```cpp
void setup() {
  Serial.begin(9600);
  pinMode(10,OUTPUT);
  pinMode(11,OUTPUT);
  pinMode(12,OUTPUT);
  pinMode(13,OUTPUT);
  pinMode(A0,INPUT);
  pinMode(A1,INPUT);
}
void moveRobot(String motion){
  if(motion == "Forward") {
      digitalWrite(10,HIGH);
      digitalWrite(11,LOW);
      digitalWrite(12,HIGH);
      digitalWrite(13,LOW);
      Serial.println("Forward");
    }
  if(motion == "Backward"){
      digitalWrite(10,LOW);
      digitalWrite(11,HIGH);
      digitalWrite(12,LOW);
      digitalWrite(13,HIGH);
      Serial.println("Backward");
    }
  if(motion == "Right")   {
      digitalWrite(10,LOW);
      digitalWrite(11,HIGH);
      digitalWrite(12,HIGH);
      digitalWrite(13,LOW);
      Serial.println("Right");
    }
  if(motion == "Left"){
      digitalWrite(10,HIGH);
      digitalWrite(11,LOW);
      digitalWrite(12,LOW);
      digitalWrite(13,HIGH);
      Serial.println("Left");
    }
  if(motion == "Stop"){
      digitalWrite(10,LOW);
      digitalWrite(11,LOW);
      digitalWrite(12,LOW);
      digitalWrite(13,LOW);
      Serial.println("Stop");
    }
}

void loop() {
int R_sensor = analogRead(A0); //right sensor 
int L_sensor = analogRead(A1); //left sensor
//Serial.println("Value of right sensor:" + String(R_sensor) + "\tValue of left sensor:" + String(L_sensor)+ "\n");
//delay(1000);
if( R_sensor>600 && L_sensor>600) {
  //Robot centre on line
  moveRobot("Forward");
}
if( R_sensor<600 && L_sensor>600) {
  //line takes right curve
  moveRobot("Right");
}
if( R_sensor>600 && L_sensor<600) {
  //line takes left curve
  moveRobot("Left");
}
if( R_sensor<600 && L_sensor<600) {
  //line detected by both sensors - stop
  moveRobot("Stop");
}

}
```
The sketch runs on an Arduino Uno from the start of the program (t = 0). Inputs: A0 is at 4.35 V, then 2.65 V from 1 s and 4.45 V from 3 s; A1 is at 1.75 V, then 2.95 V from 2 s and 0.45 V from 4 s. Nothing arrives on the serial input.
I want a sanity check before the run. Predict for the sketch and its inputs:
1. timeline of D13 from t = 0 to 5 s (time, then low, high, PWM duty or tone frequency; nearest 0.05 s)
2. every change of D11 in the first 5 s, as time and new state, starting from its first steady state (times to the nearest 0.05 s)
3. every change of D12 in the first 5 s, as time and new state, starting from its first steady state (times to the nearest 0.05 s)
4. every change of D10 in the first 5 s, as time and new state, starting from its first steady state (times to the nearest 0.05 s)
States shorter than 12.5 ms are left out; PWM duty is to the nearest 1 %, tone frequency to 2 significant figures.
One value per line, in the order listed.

0 s high; 1 s low; 4 s high
0 s low; 2 s high; 3 s low
0 s low; 2 s high; 4 s low
0 s high; 1 s low; 3 s high
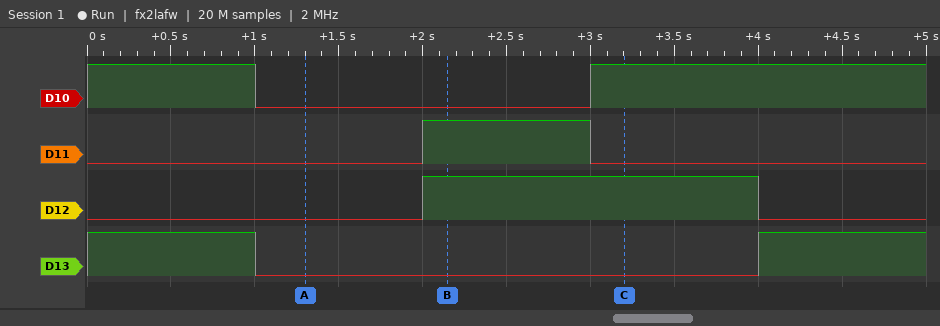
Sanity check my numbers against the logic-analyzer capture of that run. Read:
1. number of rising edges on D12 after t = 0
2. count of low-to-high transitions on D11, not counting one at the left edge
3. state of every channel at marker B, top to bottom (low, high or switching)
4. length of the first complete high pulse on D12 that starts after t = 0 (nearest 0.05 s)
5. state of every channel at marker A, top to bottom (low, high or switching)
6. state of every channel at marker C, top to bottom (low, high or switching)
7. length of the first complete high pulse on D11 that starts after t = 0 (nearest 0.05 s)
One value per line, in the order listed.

1
1
D10 low, D11 high, D12 high, D13 low
2.00 s
D10 low, D11 low, D12 low, D13 low
D10 high, D11 low, D12 high, D13 low
1.00 s
